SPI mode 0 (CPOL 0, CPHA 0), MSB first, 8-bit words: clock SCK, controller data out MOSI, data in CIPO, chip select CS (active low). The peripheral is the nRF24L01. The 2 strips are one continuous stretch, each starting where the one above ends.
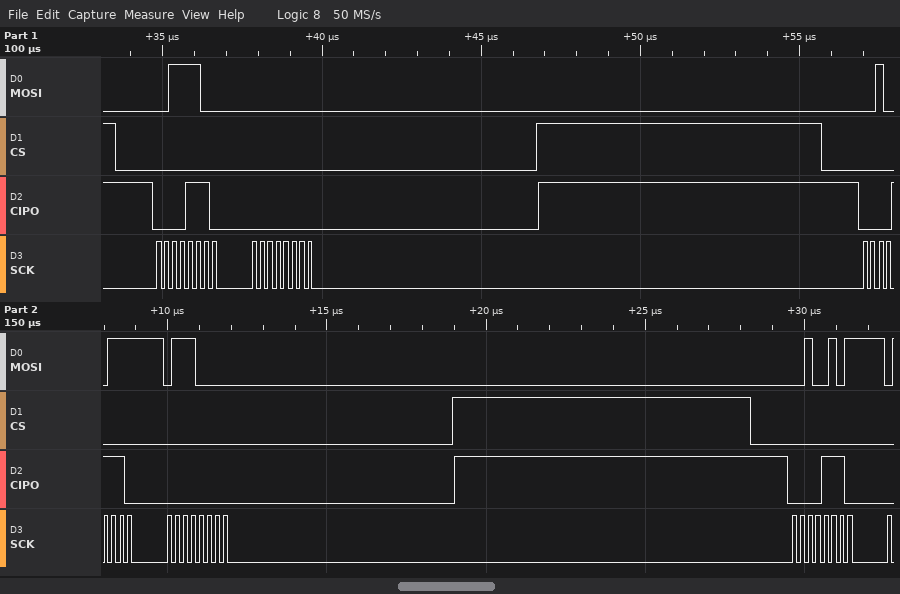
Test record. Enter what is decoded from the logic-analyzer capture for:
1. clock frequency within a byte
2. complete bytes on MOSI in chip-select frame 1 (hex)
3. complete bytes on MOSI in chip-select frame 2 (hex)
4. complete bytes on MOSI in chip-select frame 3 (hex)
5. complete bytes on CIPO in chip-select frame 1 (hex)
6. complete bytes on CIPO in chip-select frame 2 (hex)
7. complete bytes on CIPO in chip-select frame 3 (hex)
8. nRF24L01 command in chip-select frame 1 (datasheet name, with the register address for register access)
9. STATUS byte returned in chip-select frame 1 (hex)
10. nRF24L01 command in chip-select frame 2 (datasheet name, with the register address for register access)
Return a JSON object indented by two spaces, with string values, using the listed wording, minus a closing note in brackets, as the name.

{
  "clock frequency within a byte": "4 MHz",
  "complete bytes on MOSI in chip-select frame 1": "3C 00",
  "complete bytes on MOSI in chip-select frame 2": "27 70",
  "complete bytes on MOSI in chip-select frame 3": "25",
  "complete bytes on CIPO in chip-select frame 1": "0E 00",
  "complete bytes on CIPO in chip-select frame 2": "0E 00",
  "complete bytes on CIPO in chip-select frame 3": "0E",
  "nRF24L01 command in chip-select frame 1": "W_REGISTER 0x1C",
  "STATUS byte returned in chip-select frame 1": "0x0E",
  "nRF24L01 command in chip-select frame 2": "W_REGISTER 0x07"
}
